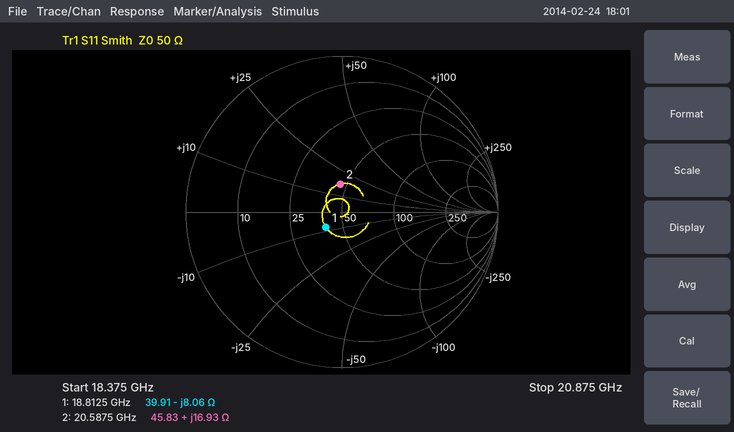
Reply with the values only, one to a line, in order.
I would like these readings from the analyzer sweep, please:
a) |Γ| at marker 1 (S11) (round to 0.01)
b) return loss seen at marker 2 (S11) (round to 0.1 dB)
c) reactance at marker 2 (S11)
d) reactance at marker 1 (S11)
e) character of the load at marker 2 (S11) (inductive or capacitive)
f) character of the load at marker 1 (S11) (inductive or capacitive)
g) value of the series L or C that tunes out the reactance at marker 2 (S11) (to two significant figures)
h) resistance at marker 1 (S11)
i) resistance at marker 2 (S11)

0.14
14.9 dB
+16.93 Ω
-8.06 Ω
inductive
capacitive
460 fF
39.91 Ω
45.83 Ω
